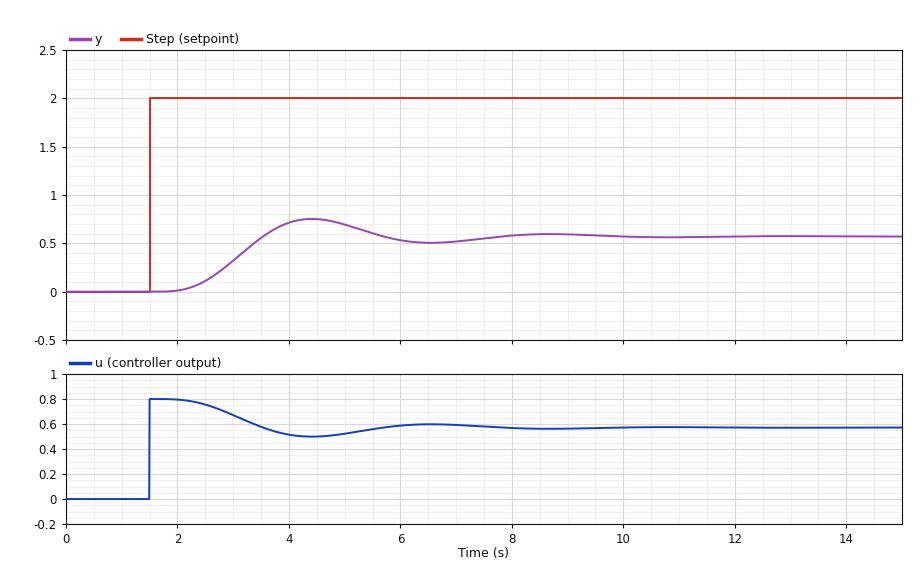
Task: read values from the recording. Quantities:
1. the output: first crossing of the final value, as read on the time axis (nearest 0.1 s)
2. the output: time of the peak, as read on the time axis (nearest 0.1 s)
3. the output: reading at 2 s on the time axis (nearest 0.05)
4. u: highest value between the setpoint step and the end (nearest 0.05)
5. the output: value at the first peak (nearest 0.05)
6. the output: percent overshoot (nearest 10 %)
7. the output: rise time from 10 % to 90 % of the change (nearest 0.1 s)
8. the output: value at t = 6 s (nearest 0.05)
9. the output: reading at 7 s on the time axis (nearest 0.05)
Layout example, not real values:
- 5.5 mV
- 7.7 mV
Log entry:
- 3.5 s
- 4.4 s
- 0.00
- 0.80
- 0.75
- 30 %
- 1.1 s
- 0.55
- 0.50
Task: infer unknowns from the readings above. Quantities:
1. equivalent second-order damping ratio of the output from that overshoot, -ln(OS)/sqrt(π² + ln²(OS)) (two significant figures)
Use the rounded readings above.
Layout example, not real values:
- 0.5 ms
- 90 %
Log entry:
- 0.36
